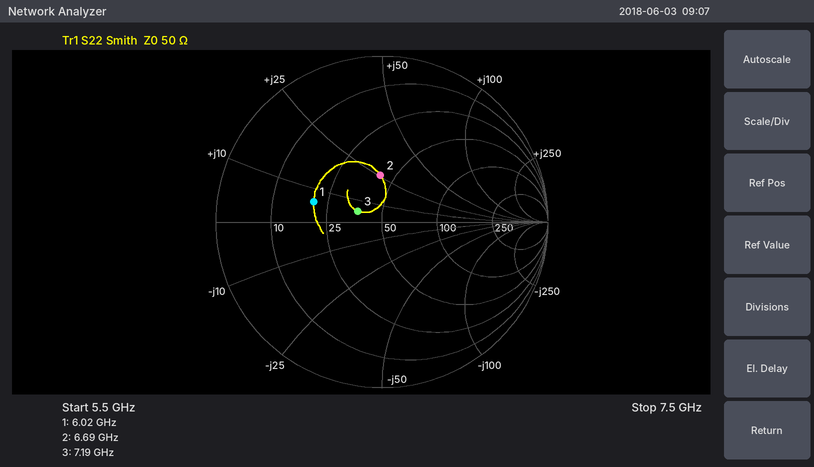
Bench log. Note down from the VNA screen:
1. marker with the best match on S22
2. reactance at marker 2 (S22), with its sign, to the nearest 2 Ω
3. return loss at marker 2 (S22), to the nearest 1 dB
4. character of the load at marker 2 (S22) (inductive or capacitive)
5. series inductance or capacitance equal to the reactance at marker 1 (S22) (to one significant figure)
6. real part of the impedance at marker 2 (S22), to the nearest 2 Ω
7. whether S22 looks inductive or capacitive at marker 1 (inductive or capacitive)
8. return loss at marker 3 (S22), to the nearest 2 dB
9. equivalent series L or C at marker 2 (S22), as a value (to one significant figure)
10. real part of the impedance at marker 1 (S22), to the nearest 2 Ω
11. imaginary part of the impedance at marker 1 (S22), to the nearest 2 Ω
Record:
marker 3
+26 Ω
11 dB
inductive
200 pH
42 Ω
inductive
16 dB
600 pH
20 Ω
+6 Ω
